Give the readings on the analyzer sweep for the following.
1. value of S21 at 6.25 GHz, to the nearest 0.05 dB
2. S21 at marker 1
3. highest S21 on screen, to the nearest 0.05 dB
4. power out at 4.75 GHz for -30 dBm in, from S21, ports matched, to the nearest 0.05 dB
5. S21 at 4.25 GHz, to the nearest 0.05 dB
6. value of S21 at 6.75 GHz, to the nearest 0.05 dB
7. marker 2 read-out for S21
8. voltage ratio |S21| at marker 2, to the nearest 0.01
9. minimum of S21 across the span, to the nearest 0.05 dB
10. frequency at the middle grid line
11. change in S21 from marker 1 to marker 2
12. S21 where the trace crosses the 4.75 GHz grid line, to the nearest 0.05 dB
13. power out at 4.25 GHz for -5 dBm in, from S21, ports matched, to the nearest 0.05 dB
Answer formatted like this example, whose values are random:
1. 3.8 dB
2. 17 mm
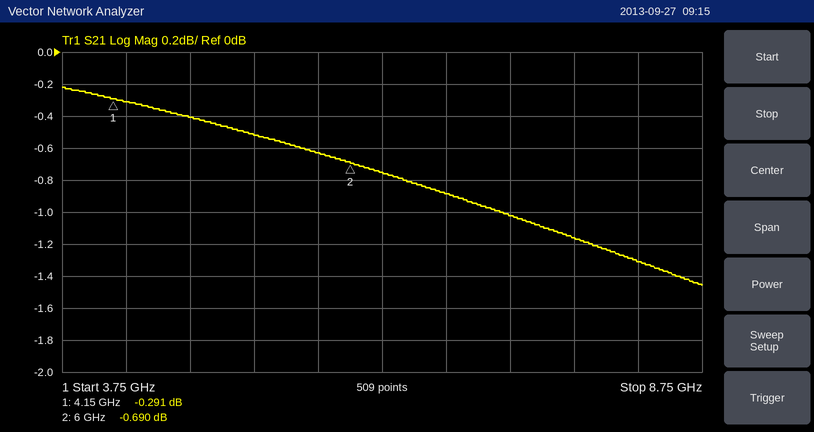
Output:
1. -0.75 dB
2. -0.291 dB
3. -0.20 dB
4. -30.40 dBm
5. -0.30 dB
6. -0.90 dB
7. -0.690 dB
8. 0.92
9. -1.45 dB
10. 6.25 GHz
11. -0.399 dB
12. -0.40 dB
13. -5.30 dBm
